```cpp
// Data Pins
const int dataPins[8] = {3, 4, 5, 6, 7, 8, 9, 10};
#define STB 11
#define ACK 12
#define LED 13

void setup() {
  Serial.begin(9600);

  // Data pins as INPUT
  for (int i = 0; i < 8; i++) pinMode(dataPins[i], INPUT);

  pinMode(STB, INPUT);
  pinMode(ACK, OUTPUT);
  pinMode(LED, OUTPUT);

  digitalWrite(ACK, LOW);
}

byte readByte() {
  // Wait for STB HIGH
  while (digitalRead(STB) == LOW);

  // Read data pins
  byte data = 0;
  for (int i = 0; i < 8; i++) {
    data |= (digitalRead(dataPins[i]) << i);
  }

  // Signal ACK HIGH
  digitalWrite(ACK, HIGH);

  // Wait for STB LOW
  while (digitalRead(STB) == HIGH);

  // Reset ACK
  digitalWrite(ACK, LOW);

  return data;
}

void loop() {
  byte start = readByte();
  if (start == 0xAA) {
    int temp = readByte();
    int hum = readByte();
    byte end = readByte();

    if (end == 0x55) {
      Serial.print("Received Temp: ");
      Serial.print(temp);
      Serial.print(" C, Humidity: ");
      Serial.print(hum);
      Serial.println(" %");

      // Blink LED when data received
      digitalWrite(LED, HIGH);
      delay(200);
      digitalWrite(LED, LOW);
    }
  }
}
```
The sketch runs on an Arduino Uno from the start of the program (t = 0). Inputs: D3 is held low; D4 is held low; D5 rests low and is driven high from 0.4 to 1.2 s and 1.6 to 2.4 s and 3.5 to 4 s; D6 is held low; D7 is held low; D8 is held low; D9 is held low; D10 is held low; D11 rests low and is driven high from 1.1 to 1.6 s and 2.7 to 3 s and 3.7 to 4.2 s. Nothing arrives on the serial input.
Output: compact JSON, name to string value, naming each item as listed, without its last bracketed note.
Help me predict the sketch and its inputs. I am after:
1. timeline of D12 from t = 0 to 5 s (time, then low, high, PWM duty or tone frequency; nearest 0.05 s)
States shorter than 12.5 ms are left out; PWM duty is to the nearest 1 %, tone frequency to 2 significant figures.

{"timeline of D12 from t = 0 to 5 s": "0 s low; 1.1 s high; 1.6 s low; 2.7 s high; 3 s low; 3.7 s high; 4.2 s low"}
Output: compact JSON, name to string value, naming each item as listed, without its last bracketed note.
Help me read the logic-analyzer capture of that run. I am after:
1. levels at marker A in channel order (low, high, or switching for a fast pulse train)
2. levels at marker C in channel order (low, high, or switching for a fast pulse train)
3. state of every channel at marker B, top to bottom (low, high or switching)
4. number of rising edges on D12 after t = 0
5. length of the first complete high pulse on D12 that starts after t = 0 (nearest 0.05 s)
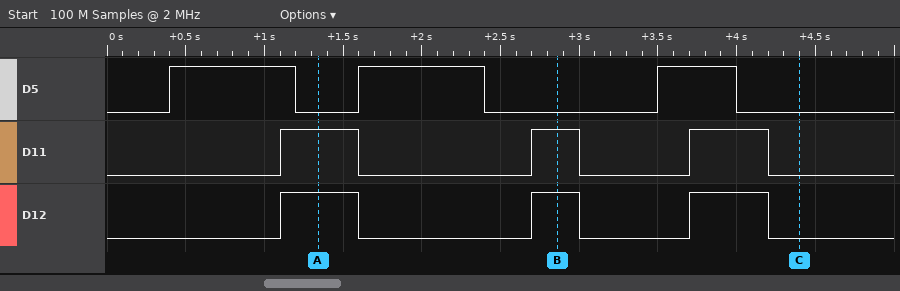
{"levels at marker A in channel order": "D5 low, D11 high, D12 high", "levels at marker C in channel order": "D5 low, D11 low, D12 low", "state of every channel at marker B, top to bottom": "D5 low, D11 high, D12 high", "number of rising edges on D12 after t = 0": "3", "length of the first complete high pulse on D12 that starts after t = 0": "0.50 s"}
